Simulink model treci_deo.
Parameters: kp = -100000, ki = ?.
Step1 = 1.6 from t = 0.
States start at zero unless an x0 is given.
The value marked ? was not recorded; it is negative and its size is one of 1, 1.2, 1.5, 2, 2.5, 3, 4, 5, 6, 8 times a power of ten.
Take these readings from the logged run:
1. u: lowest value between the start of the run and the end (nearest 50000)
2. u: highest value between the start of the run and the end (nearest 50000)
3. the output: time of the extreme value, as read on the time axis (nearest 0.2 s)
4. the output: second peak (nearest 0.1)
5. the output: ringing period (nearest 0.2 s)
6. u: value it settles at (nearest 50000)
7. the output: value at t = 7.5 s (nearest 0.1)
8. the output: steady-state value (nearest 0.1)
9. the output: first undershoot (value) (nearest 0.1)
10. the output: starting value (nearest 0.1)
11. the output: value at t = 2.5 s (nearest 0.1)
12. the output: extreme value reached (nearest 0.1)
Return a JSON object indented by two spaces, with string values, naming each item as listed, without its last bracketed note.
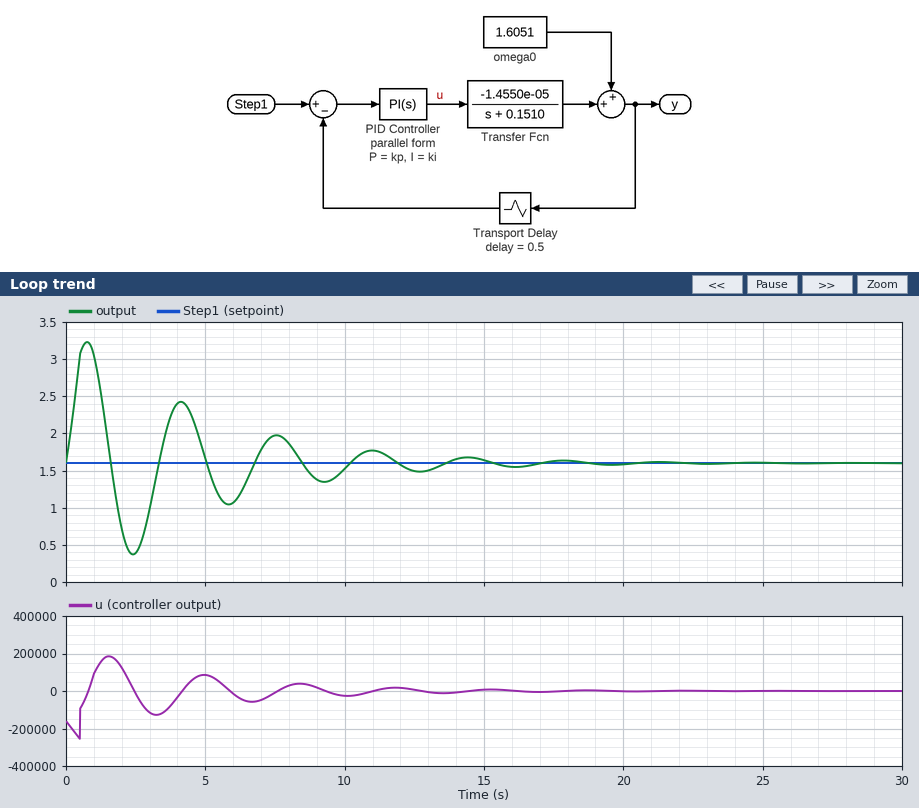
{
  "u: lowest value between the start of the run and the end": "-250000",
  "u: highest value between the start of the run and the end": "200000",
  "the output: time of the extreme value, as read on the time axis": "0.8 s",
  "the output: second peak": "2.4",
  "the output: ringing period": "3.4 s",
  "u: value it settles at": "0",
  "the output: value at t = 7.5 s": "2.0",
  "the output: steady-state value": "1.6",
  "the output: first undershoot (value)": "0.4",
  "the output: starting value": "1.6",
  "the output: value at t = 2.5 s": "0.4",
  "the output: extreme value reached": "3.2"
}
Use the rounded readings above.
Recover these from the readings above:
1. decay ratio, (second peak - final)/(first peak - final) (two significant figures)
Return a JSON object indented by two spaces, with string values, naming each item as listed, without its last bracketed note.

{
  "decay ratio, (second peak - final)/(first peak - final)": "0.50"
}
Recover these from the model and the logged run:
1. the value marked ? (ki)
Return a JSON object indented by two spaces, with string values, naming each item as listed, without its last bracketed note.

{
  "the value marked ?": "-120000"
}
